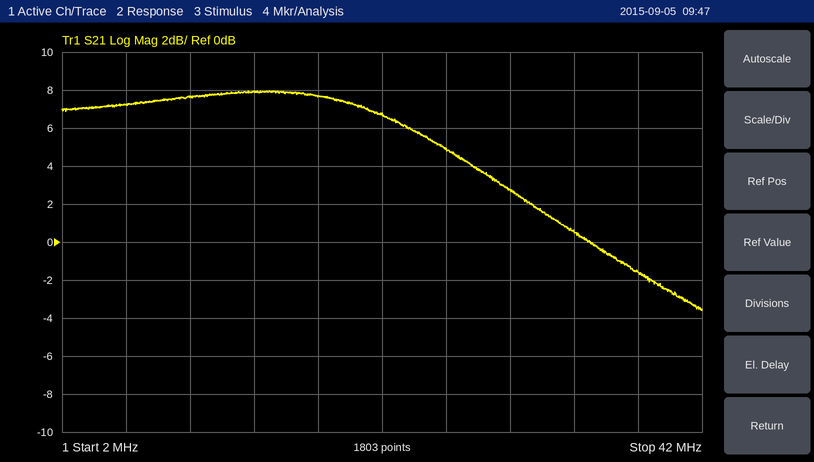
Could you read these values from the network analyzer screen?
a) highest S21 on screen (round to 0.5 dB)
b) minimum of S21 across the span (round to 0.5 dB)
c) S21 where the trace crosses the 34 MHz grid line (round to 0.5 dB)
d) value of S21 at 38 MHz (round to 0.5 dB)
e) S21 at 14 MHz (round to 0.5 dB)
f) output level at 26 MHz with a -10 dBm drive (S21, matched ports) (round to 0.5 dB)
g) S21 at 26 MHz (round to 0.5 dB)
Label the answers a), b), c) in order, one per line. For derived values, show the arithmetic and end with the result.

a) 8.0 dB
b) -3.5 dB
c) 0.5 dB
d) -1.5 dB
e) 8.0 dB
f) -10 dBm + (5.0 dB) = -5.0 dBm
g) 5.0 dB
